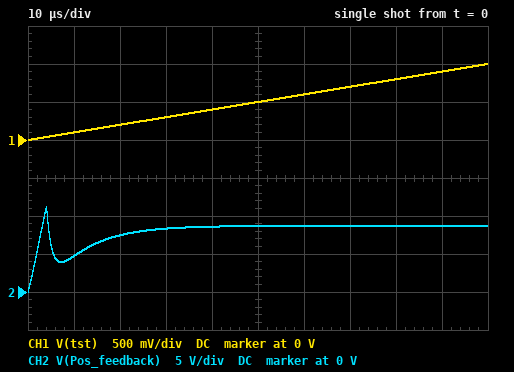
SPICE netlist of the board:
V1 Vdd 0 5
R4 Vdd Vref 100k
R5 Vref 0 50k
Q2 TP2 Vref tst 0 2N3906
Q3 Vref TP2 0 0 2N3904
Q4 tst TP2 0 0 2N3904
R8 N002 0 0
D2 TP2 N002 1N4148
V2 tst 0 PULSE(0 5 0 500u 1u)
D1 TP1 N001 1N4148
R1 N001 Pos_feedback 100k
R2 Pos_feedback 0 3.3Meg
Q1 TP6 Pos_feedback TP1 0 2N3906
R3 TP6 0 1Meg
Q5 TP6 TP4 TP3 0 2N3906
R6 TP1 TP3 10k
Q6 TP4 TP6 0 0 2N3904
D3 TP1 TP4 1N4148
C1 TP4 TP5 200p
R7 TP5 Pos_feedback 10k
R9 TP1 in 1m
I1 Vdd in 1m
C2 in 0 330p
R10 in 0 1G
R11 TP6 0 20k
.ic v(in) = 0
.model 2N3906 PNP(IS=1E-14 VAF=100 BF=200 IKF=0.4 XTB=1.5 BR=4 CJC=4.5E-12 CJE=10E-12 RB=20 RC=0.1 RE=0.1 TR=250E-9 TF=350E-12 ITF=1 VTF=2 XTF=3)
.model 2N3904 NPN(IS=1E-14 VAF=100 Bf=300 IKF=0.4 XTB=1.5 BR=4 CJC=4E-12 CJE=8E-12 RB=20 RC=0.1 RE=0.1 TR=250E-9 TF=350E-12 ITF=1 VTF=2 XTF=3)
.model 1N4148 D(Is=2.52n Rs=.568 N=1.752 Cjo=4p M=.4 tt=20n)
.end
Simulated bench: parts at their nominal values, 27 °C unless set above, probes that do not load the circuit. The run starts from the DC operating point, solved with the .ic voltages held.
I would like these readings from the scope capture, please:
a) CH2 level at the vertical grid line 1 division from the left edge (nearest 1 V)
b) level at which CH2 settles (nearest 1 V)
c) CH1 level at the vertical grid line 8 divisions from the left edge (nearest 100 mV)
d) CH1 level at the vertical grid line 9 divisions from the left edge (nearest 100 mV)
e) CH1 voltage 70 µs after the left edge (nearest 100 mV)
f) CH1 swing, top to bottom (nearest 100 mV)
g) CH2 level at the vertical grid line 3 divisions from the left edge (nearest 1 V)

5 V
9 V
800 mV
900 mV
700 mV
1.0 V
8 V
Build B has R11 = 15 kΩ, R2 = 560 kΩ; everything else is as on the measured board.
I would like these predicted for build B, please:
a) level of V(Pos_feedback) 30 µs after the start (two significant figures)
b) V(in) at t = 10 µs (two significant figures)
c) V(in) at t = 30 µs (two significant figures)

1.6 V
2.0 V
2.1 V
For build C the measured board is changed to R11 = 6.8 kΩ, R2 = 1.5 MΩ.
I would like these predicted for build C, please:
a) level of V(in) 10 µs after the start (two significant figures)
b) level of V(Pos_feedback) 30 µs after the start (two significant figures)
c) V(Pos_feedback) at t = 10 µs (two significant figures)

4.3 V
4.8 V
3.7 V
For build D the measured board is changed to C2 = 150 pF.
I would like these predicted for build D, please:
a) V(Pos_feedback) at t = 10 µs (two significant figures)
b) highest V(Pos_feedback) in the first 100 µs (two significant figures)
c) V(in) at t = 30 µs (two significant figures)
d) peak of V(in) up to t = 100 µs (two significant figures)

6.3 V
8.7 V
9.1 V
9.3 V
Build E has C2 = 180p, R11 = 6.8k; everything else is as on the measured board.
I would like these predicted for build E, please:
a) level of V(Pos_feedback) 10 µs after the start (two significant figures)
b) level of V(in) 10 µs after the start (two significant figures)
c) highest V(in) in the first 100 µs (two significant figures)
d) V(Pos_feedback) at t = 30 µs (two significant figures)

8.2 V
8.8 V
11 V
10 V
